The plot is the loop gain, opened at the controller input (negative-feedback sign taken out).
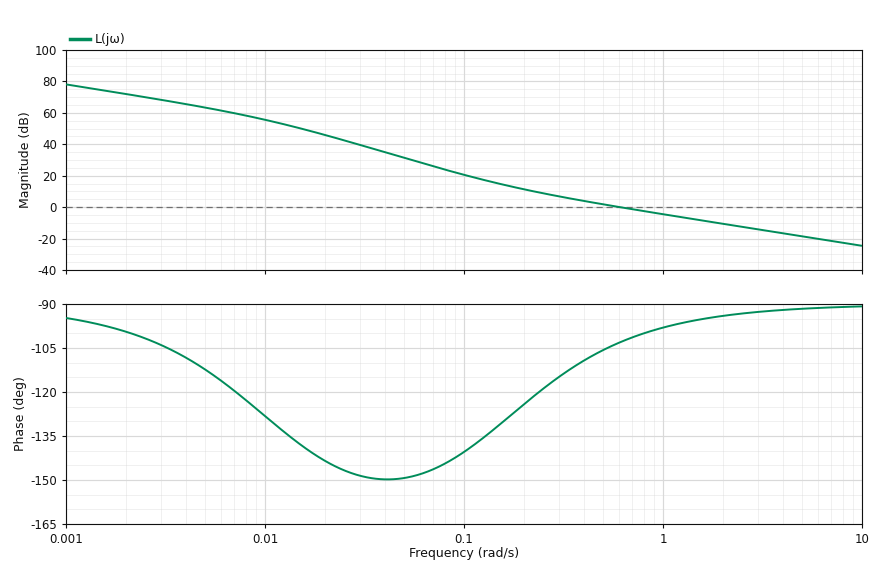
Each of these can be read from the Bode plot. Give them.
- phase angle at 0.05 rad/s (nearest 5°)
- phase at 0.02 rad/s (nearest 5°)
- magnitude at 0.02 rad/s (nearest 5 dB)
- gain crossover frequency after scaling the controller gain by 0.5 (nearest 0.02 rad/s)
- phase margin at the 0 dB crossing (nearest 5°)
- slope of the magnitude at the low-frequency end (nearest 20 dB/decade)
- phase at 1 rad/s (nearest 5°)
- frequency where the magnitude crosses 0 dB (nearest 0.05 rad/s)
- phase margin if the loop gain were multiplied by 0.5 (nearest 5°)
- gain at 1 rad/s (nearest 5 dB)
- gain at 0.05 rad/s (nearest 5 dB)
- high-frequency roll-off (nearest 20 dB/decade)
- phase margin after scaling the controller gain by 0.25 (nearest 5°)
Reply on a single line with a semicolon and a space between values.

-150°; -145°; 45 dB; 0.32 rad/s; 75°; -20 dB/decade; -100°; 0.60 rad/s; 65°; -5 dB; 30 dB; -20 dB/decade; 55°
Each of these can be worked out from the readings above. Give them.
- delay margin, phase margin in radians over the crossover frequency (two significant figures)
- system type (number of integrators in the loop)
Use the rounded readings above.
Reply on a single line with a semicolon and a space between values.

2.2 s; 1
